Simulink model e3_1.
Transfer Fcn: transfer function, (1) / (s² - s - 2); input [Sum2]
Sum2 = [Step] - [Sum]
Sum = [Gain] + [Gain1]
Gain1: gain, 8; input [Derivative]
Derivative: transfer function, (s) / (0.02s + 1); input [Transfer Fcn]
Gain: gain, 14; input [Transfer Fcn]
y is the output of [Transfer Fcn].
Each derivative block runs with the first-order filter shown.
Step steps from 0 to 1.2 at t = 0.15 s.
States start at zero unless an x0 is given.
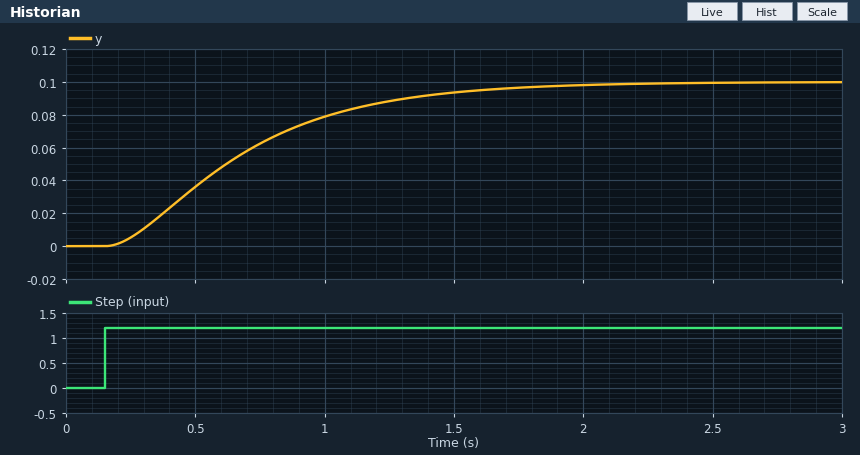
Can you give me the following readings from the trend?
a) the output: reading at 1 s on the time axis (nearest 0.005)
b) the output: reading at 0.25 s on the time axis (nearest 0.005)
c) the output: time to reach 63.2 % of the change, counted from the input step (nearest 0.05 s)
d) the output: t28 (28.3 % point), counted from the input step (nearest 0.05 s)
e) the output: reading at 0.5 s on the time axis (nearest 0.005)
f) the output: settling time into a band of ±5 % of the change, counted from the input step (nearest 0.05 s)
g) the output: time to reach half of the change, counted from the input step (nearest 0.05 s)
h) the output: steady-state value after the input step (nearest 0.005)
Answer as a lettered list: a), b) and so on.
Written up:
a) 0.080
b) 0.005
c) 0.60 s
d) 0.30 s
e) 0.035
f) 1.45 s
g) 0.45 s
h) 0.100
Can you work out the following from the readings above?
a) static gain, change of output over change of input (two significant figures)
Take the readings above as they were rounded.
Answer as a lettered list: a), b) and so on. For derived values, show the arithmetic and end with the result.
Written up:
a) (0.1 - 0) / (1.2 - 0) = 0.083
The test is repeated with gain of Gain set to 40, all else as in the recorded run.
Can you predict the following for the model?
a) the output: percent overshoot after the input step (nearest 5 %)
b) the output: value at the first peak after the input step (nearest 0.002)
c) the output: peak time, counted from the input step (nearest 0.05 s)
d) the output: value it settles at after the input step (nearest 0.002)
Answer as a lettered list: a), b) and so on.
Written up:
a) 10 %
b) 0.034
c) 0.60 s
d) 0.032
